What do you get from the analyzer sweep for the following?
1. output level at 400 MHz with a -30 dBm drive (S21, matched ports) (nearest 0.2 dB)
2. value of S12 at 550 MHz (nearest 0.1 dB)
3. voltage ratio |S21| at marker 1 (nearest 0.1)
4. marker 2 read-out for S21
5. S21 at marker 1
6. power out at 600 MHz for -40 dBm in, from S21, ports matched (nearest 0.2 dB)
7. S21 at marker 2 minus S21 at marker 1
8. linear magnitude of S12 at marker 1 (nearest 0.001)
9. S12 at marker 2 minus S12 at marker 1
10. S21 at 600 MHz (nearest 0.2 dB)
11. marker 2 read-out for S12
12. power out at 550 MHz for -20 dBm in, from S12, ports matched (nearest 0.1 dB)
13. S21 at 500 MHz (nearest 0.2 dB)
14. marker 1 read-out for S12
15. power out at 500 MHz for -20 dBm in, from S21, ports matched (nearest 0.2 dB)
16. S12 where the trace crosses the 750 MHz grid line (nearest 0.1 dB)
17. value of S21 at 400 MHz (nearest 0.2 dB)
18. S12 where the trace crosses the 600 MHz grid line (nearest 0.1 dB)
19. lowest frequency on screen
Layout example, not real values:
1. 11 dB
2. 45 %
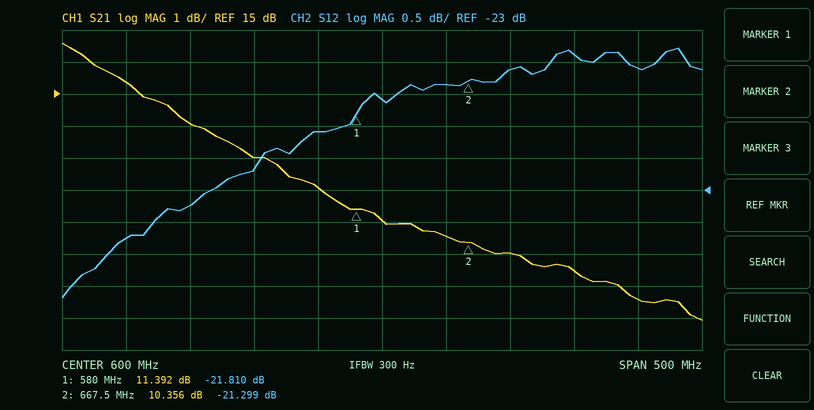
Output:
1. -14.6 dBm
2. -22.1 dB
3. 3.7
4. 10.356 dB
5. 11.392 dB
6. -29.0 dBm
7. -1.036 dB
8. 0.081
9. 0.511 dB
10. 11.0 dB
11. -21.299 dB
12. -42.1 dBm
13. 13.0 dB
14. -21.810 dB
15. -7.0 dBm
16. -20.9 dB
17. 15.4 dB
18. -21.6 dB
19. 350 MHz
